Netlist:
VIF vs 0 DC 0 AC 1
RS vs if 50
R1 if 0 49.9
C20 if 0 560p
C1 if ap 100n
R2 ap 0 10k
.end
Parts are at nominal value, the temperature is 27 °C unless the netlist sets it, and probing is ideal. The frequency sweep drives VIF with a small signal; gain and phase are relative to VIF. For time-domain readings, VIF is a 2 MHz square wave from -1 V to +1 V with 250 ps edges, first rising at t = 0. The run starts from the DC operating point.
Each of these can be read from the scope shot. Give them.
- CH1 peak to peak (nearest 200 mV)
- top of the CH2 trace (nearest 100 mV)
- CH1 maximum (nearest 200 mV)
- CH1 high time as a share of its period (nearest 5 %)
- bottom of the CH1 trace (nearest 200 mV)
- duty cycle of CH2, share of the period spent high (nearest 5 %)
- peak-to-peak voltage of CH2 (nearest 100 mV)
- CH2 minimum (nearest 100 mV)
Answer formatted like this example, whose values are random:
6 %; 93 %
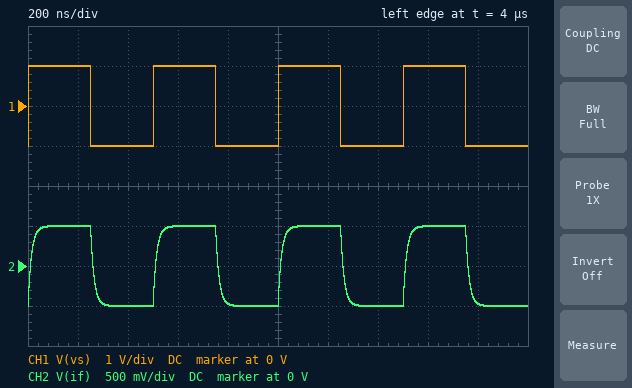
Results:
2.0 V; 500 mV; 1.0 V; 50 %; -1.0 V; 50 %; 1.0 V; -500 mV
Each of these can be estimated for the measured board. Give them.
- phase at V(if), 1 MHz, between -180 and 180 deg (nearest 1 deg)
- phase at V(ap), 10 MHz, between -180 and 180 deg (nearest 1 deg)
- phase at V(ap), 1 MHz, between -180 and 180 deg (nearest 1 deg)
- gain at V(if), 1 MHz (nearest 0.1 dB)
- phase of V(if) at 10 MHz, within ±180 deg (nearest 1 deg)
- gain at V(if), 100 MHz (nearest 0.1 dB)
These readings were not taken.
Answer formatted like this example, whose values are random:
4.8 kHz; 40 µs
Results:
-5 deg; -41 deg; -5 deg; -6.1 dB; -41 deg; -25.0 dB
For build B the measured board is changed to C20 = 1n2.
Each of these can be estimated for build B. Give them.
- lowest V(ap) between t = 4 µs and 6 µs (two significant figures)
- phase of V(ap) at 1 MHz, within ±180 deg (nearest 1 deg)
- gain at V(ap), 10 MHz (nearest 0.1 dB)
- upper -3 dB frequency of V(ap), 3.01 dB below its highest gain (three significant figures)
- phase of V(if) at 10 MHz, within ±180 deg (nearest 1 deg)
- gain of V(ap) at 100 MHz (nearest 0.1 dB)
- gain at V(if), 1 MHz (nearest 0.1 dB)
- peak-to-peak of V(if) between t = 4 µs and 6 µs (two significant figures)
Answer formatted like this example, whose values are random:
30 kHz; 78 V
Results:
-2.7 mV; -11 deg; -12.6 dB; 5.32 MHz; -62 deg; -31.5 dB; -6.2 dB; 1.0 V
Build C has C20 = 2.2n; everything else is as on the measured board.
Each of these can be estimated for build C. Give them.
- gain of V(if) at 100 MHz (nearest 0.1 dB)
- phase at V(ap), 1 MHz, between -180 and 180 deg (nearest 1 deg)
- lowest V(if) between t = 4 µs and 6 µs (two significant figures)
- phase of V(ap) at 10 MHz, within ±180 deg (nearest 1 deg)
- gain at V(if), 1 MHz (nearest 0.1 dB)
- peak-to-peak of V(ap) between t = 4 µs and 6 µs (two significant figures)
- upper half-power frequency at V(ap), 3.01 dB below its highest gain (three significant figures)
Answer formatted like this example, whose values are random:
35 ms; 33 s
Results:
-36.8 dB; -19 deg; -490 mV; -74 deg; -6.5 dB; 980 mV; 2.90 MHz
